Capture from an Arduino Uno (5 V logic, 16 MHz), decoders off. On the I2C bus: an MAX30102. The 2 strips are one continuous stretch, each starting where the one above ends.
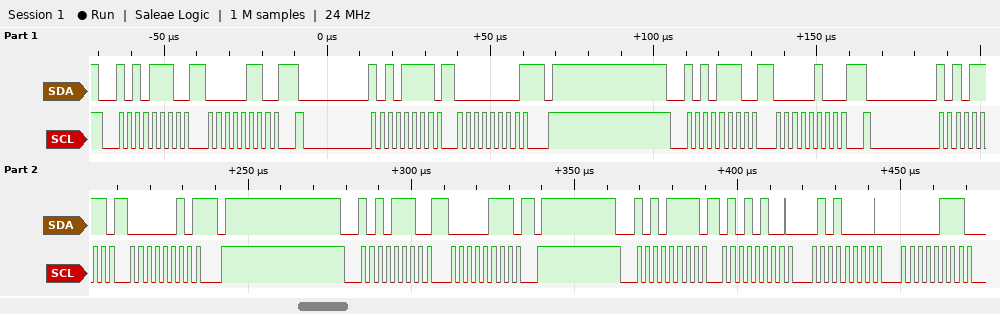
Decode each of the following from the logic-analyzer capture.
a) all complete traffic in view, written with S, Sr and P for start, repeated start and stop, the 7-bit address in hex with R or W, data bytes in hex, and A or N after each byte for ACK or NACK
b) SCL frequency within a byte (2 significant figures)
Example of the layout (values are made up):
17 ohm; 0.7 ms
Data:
S 57W A 06 A Sr 57R A 00 N P S 57W A 04 A Sr 57R A 02 N P S 57W A 07 A P S 57R A 54 A 50 A 07 A; 400 kHz
